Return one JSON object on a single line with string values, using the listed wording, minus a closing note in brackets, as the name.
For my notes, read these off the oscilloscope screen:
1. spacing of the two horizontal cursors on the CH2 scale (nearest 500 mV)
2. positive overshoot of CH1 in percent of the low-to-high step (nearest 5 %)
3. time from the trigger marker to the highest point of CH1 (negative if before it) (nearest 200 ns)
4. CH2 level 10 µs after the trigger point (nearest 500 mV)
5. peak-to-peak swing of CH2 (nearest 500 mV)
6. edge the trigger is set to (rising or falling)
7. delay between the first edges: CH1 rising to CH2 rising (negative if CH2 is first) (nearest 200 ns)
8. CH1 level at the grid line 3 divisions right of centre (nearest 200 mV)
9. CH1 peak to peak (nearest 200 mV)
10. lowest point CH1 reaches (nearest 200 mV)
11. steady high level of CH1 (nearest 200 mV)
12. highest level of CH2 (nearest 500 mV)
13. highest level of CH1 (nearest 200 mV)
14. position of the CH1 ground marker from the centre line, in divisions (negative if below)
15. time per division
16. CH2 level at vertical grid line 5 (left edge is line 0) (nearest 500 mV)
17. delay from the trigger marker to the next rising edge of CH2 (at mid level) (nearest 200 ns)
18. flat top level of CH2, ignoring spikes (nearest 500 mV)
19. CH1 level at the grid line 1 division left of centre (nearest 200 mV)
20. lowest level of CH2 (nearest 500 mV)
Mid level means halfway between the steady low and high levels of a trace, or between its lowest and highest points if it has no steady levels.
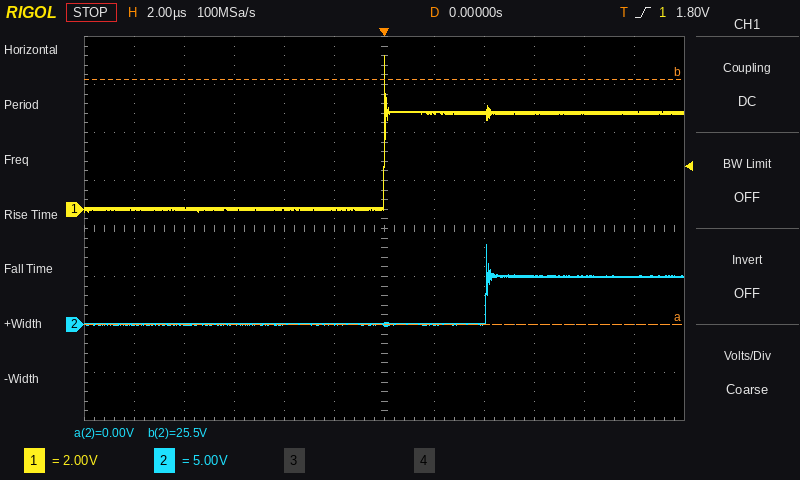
{"spacing of the two horizontal cursors on the CH2 scale": "25.5 V", "positive overshoot of CH1 in percent of the low-to-high step": "60 %", "time from the trigger marker to the highest point of CH1 (negative if before it)": "0.0 µs", "CH2 level 10 µs after the trigger point": "5.0 V", "peak-to-peak swing of CH2": "8.5 V", "edge the trigger is set to": "rising", "delay between the first edges: CH1 rising to CH2 rising (negative if CH2 is first)": "+4.0 µs", "CH1 level at the grid line 3 divisions right of centre": "4.0 V", "CH1 peak to peak": "6.4 V", "lowest point CH1 reaches": "0.0 V", "steady high level of CH1": "4.0 V", "highest level of CH2": "8.5 V", "highest level of CH1": "6.4 V", "position of the CH1 ground marker from the centre line, in divisions": "+0.4 div", "time per division": "2 µs", "CH2 level at vertical grid line 5 (left edge is line 0)": "0.0 V", "delay from the trigger marker to the next rising edge of CH2 (at mid level)": "4.0 µs", "flat top level of CH2, ignoring spikes": "5.0 V", "CH1 level at the grid line 1 division left of centre": "0.0 V", "lowest level of CH2": "0.0 V"}
